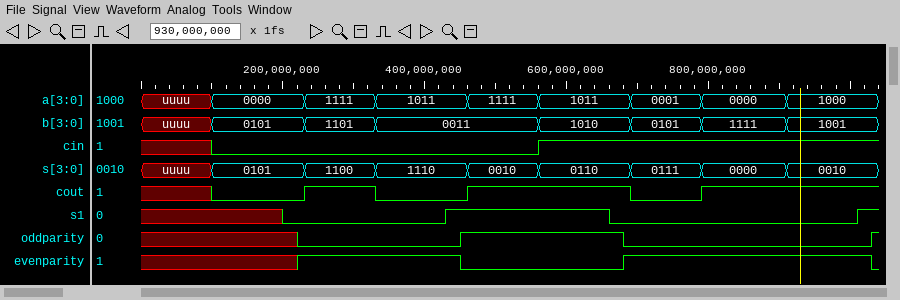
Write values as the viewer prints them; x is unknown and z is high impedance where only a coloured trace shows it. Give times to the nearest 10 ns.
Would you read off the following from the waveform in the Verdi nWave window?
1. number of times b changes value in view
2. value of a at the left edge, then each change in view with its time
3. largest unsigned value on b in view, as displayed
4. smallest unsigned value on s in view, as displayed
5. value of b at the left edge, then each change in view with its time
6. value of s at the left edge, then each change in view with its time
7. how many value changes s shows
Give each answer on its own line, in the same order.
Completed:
7
uuuu, 0000 at 100 ns, 1111 at 230 ns, 1011 at 330 ns, 1111 at 460 ns, 1011 at 560 ns, 0001 at 690 ns, 0000 at 790 ns, 1000 at 910 ns
1111
0000
uuuu, 0101 at 100 ns, 1101 at 230 ns, 0011 at 330 ns, 1010 at 560 ns, 0101 at 690 ns, 1111 at 790 ns, 1001 at 910 ns
uuuu, 0101 at 100 ns, 1100 at 230 ns, 1110 at 330 ns, 0010 at 460 ns, 0110 at 560 ns, 0111 at 690 ns, 0000 at 790 ns, 0010 at 910 ns
8
